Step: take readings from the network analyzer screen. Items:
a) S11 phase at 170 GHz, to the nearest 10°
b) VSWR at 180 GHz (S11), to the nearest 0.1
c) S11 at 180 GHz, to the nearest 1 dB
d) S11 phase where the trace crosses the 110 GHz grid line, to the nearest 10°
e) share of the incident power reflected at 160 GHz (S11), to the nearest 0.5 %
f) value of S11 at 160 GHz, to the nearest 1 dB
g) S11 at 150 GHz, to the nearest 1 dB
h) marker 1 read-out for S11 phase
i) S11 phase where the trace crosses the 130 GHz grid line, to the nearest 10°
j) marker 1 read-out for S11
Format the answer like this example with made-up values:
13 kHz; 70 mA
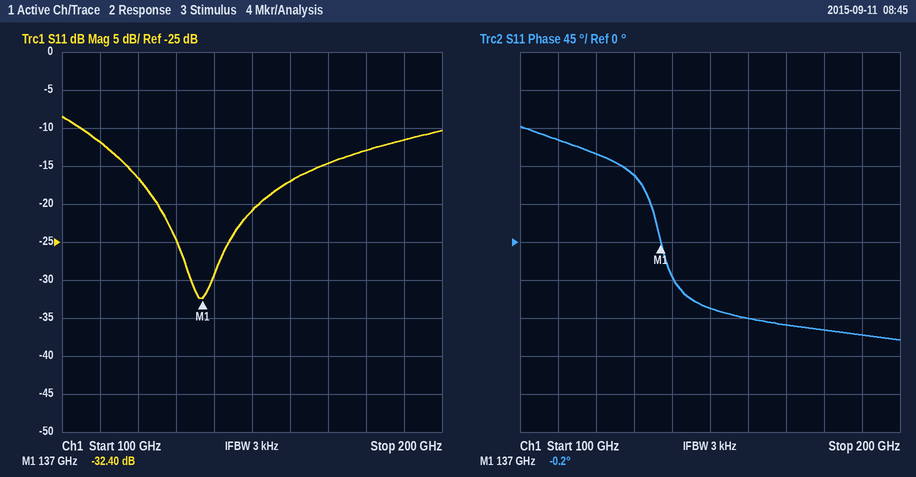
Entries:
-100°; 1.6; -13 dB; 120°; 2.0 %; -17 dB; -21 dB; -0.2°; 80°; -32.40 dB
